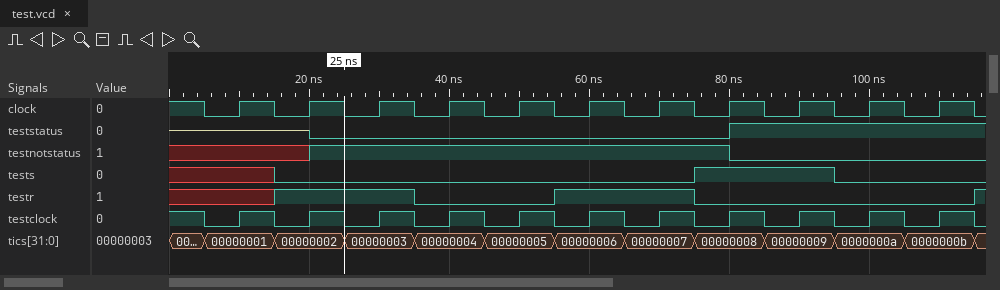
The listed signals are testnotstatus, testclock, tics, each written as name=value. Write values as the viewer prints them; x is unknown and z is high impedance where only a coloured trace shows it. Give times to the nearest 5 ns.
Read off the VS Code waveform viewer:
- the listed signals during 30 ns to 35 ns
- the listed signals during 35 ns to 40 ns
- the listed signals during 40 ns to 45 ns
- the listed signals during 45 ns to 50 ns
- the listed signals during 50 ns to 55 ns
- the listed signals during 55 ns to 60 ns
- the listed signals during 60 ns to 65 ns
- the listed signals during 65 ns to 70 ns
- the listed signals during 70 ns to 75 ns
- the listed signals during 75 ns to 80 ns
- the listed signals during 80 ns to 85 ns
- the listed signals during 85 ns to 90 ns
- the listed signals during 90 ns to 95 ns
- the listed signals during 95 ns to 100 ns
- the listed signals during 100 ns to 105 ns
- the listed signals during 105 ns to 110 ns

testnotstatus=1, testclock=1, tics=00000003
testnotstatus=1, testclock=0, tics=00000004
testnotstatus=1, testclock=1, tics=00000004
testnotstatus=1, testclock=0, tics=00000005
testnotstatus=1, testclock=1, tics=00000005
testnotstatus=1, testclock=0, tics=00000006
testnotstatus=1, testclock=1, tics=00000006
testnotstatus=1, testclock=0, tics=00000007
testnotstatus=1, testclock=1, tics=00000007
testnotstatus=1, testclock=0, tics=00000008
testnotstatus=0, testclock=1, tics=00000008
testnotstatus=0, testclock=0, tics=00000009
testnotstatus=0, testclock=1, tics=00000009
testnotstatus=0, testclock=0, tics=0000000a
testnotstatus=0, testclock=1, tics=0000000a
testnotstatus=0, testclock=0, tics=0000000b
